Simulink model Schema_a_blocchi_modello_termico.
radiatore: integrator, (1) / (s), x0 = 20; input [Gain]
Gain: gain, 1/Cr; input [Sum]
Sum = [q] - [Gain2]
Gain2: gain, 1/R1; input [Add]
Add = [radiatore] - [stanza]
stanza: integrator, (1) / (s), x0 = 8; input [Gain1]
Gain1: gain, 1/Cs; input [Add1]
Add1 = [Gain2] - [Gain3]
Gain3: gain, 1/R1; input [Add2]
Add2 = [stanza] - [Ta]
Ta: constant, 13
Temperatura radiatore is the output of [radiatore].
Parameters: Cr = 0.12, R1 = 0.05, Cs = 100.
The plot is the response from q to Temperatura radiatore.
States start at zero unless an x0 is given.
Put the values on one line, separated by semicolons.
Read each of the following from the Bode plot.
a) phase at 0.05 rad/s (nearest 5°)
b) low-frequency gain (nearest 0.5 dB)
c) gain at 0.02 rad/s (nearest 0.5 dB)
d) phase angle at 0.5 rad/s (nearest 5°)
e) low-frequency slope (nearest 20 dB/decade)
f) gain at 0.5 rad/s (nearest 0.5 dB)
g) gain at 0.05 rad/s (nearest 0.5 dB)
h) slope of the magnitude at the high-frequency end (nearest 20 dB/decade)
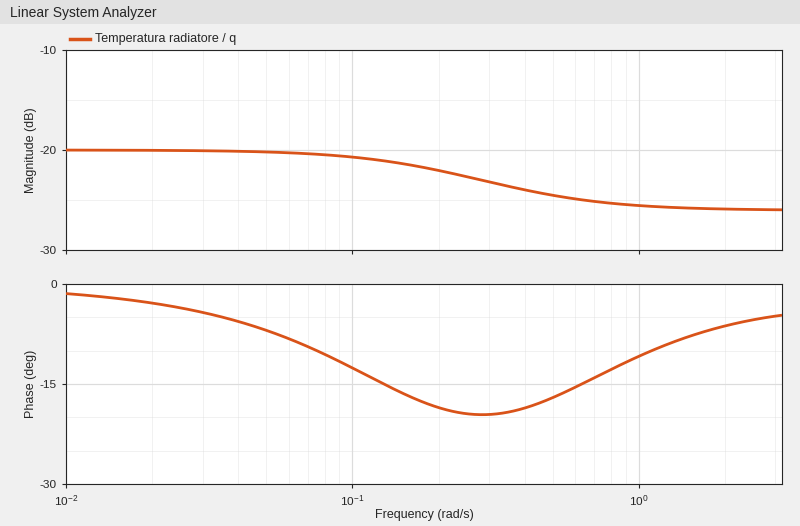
-5°; -20.0 dB; -20.0 dB; -15°; 0 dB/decade; -24.5 dB; -20.0 dB; 0 dB/decade
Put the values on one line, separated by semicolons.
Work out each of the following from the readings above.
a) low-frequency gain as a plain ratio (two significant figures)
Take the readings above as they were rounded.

0.10
